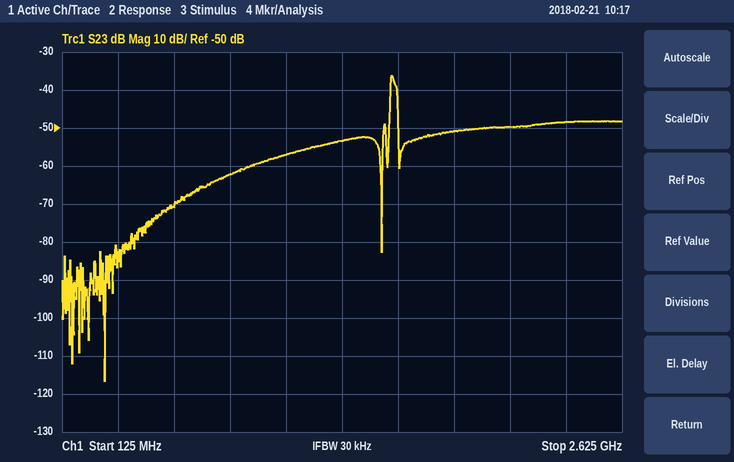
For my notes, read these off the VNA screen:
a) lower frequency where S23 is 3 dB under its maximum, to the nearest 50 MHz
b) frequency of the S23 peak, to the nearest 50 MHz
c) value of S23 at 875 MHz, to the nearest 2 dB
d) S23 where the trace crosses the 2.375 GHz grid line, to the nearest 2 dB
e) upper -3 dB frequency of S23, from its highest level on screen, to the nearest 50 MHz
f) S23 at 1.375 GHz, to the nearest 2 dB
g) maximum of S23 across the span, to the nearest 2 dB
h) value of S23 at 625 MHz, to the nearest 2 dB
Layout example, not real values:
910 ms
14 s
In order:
1.60 GHz
1.60 GHz
-62 dB
-48 dB
1.60 GHz
-54 dB
-36 dB
-70 dB
